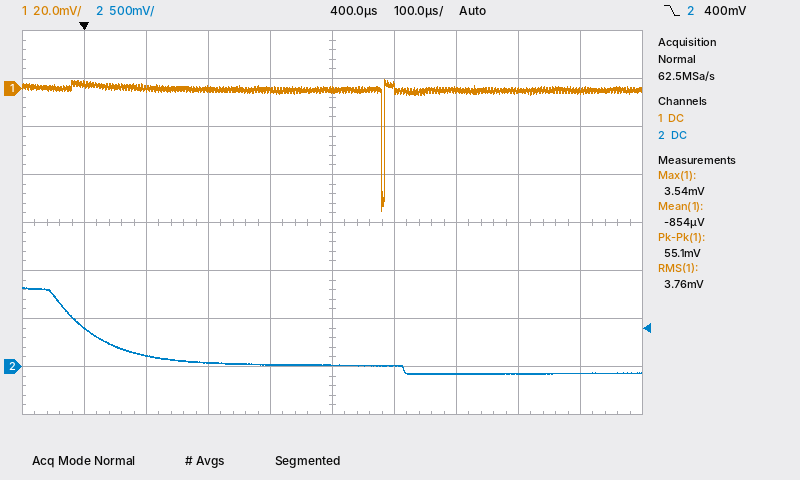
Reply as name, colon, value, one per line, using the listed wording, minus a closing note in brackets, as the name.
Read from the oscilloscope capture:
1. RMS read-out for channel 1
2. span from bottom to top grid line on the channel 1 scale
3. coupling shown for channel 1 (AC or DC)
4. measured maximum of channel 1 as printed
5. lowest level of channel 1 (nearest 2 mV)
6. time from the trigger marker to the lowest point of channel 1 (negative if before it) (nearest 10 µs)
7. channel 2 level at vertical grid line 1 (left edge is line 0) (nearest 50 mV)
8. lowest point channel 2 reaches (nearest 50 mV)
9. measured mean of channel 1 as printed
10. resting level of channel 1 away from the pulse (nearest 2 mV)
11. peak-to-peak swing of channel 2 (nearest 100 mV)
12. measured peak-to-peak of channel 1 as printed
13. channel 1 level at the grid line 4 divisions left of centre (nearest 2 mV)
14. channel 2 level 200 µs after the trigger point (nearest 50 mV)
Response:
RMS read-out for channel 1: 3.76 mV
span from bottom to top grid line on the channel 1 scale: 160 mV
coupling shown for channel 1: DC
measured maximum of channel 1 as printed: 3.54 mV
lowest level of channel 1: -52 mV
time from the trigger marker to the lowest point of channel 1 (negative if before it): +480 µs
channel 2 level at vertical grid line 1 (left edge is line 0): 400 mV
lowest point channel 2 reaches: -100 mV
measured mean of channel 1 as printed: -854 µV
resting level of channel 1 away from the pulse: 0 mV
peak-to-peak swing of channel 2: 900 mV
measured peak-to-peak of channel 1 as printed: 55.1 mV
channel 1 level at the grid line 4 divisions left of centre: 2 mV
channel 2 level 200 µs after the trigger point: 50 mV
